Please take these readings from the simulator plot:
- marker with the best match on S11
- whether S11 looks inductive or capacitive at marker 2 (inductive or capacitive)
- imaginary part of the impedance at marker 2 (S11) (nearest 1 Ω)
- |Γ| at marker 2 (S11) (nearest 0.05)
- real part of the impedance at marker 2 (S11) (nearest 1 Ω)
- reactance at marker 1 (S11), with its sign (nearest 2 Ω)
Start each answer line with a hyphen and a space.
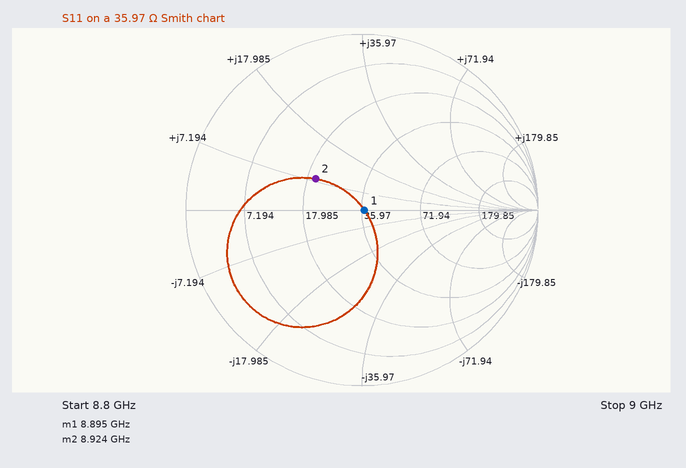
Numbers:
- marker 1
- inductive
- +8 Ω
- 0.30
- 20 Ω
- 0 Ω
